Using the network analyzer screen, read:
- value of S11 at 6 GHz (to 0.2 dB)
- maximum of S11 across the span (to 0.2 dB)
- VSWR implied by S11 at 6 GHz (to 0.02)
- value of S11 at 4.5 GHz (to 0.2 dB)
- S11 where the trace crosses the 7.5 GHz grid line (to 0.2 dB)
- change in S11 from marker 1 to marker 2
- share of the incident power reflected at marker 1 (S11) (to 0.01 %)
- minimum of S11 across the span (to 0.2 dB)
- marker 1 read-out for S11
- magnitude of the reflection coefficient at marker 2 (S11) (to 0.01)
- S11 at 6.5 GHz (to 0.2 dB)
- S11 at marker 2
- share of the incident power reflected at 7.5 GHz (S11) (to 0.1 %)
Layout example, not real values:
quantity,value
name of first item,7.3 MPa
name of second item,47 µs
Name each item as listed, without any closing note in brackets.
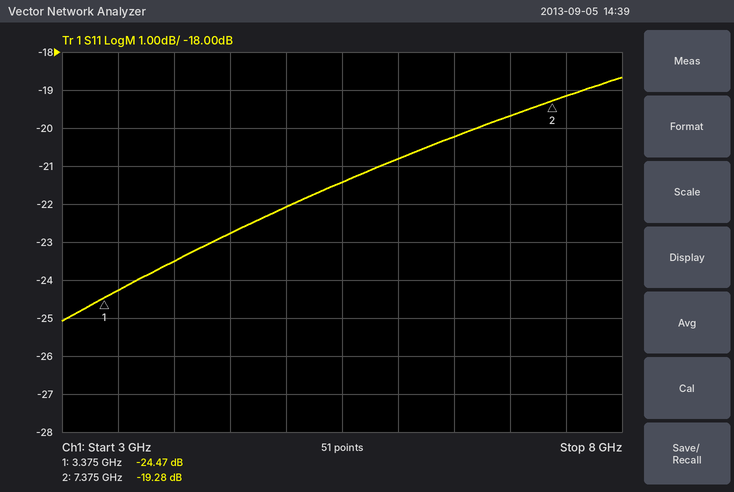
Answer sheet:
quantity,value
value of S11 at 6 GHz,-20.8 dB
maximum of S11 across the span,-18.6 dB
VSWR implied by S11 at 6 GHz,1.20
value of S11 at 4.5 GHz,-22.8 dB
S11 where the trace crosses the 7.5 GHz grid line,-19.2 dB
change in S11 from marker 1 to marker 2,5.19 dB
share of the incident power reflected at marker 1 (S11),0.36 %
minimum of S11 across the span,-25.0 dB
marker 1 read-out for S11,-24.47 dB
magnitude of the reflection coefficient at marker 2 (S11),0.11
S11 at 6.5 GHz,-20.2 dB
S11 at marker 2,-19.28 dB
share of the incident power reflected at 7.5 GHz (S11),1.2 %
